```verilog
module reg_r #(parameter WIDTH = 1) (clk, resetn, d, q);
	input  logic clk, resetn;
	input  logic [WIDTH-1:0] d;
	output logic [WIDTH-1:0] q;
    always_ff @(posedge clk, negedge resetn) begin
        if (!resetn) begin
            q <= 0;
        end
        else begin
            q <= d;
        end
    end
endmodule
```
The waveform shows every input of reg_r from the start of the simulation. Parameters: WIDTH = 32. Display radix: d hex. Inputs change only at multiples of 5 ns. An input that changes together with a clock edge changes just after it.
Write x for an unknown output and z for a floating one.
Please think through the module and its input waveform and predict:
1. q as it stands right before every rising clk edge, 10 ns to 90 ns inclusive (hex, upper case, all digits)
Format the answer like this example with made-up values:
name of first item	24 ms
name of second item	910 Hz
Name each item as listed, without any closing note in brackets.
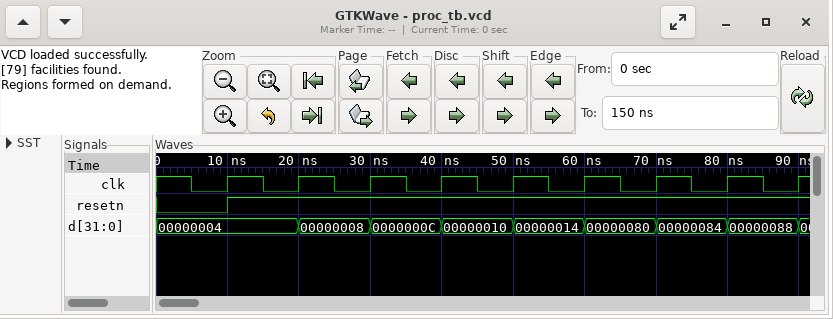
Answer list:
q as it stands right before every rising clk edge, 10 ns to 90 ns inclusive	00000000, 00000000, 00000004, 00000008, 0000000C, 00000010, 00000014, 00000080, 00000084
